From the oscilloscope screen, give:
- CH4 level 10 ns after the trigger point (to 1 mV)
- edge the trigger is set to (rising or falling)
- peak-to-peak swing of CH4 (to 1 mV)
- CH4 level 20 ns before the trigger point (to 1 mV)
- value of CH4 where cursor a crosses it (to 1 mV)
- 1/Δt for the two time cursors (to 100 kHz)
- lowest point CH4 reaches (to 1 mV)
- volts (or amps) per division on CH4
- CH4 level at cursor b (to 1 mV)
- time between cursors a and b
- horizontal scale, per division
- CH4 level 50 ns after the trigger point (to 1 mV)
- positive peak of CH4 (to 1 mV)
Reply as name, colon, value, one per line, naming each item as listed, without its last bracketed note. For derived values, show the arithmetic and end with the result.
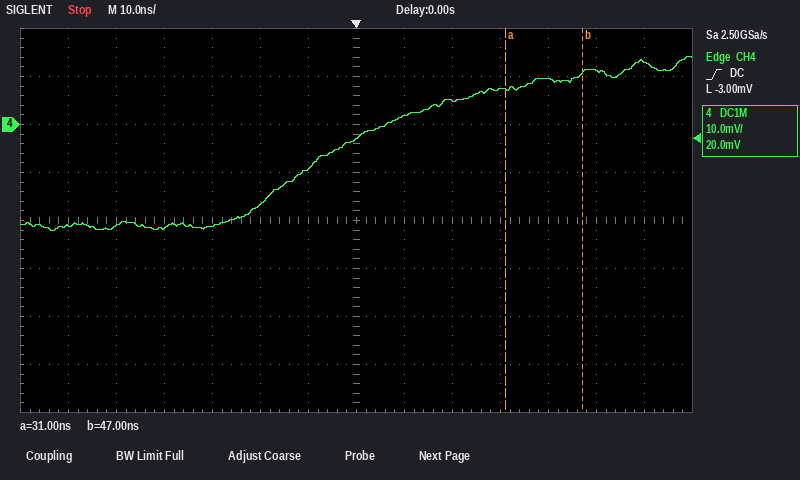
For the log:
CH4 level 10 ns after the trigger point: 2 mV
edge the trigger is set to: rising
peak-to-peak swing of CH4: 14 mV − (-22 mV) = 36 mV
CH4 level 20 ns before the trigger point: -17 mV
value of CH4 where cursor a crosses it: 7 mV
1/Δt for the two time cursors: 1 / 16 ns ≈ 62.5 MHz
lowest point CH4 reaches: -22 mV
volts (or amps) per division on CH4: 10 mV
CH4 level at cursor b: 11 mV
time between cursors a and b: 47 ns − (31 ns) = 16 ns
horizontal scale, per division: 10 ns
CH4 level 50 ns after the trigger point: 11 mV
positive peak of CH4: 14 mV
